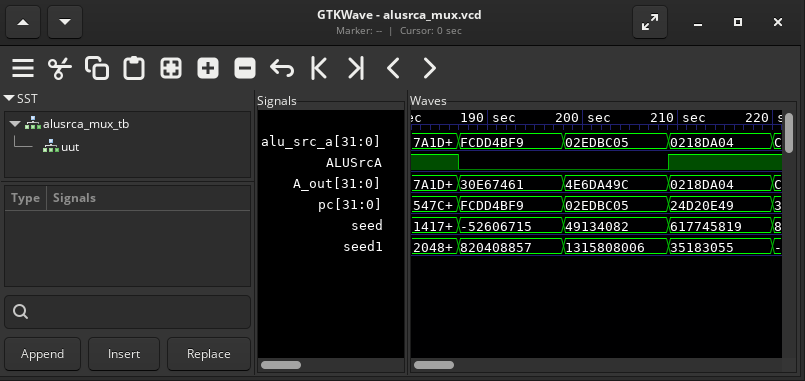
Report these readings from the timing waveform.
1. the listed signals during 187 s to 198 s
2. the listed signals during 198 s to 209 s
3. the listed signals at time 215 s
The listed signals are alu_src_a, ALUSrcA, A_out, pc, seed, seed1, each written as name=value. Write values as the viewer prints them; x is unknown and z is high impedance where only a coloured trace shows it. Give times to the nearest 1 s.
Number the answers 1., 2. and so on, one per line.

1. alu_src_a=FCDD4BF9, ALUSrcA=0, A_out=30E67461, pc=FCDD4BF9, seed=-52606715, seed1=820408857
2. alu_src_a=02EDBC05, ALUSrcA=0, A_out=4E6DA49C, pc=02EDBC05, seed=49134082, seed1=1315808006
3. alu_src_a=0218DA04, ALUSrcA=1, A_out=0218DA04, pc=24D20E49, seed=617745819, seed1=35183055
